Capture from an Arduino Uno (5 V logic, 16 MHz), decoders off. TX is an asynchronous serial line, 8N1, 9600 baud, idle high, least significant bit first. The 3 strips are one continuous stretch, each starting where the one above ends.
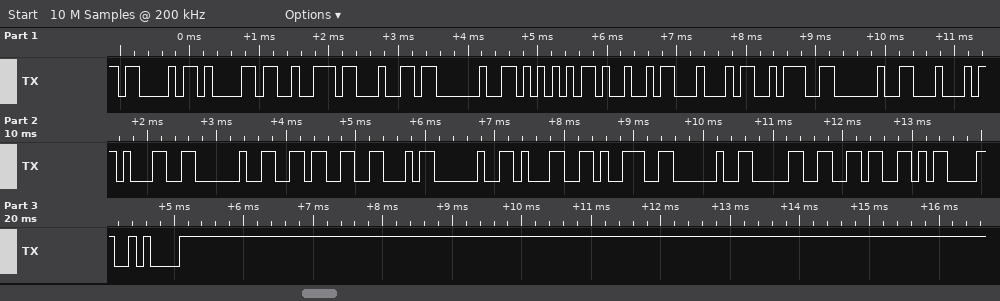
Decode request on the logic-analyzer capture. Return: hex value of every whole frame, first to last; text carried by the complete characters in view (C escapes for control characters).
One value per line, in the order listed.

43 61 72 64 20 55 49 44 3A 20 44 31 20 36 46 20 31 39 20 30 36 0D 0A
"Card UID: D1 6F 19 06\r\n"
